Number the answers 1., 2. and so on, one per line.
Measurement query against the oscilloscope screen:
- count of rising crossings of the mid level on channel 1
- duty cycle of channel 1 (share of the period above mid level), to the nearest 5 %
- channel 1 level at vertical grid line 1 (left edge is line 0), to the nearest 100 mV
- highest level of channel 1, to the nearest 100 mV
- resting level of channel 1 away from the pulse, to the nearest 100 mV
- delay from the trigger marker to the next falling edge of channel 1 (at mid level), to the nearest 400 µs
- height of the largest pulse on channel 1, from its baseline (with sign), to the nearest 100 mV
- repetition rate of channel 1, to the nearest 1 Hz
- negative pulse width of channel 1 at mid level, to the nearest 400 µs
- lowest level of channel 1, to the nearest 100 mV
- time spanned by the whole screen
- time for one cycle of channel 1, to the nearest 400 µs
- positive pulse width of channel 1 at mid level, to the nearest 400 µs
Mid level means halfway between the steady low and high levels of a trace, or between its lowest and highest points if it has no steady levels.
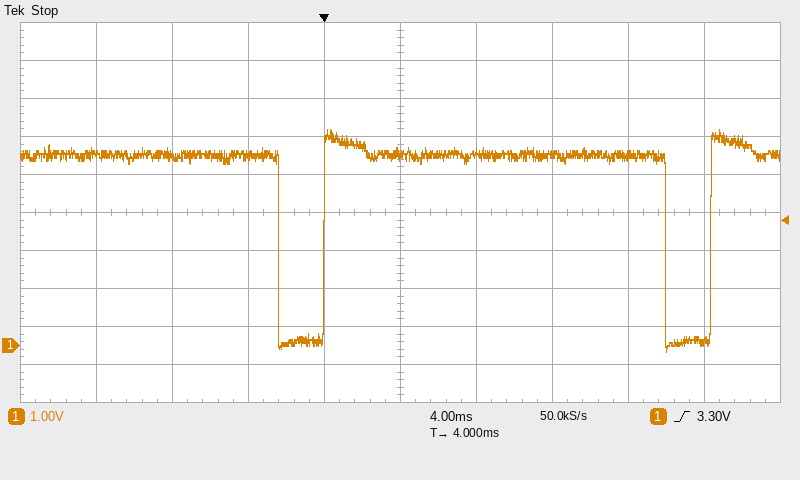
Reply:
1. 2
2. 90 %
3. 5.0 V
4. 5.7 V
5. 5.0 V
6. 18.0 ms
7. -5.2 V
8. 49 Hz
9. 2.4 ms
10. -200 mV
11. 40 ms
12. 20.4 ms
13. 18.0 ms
